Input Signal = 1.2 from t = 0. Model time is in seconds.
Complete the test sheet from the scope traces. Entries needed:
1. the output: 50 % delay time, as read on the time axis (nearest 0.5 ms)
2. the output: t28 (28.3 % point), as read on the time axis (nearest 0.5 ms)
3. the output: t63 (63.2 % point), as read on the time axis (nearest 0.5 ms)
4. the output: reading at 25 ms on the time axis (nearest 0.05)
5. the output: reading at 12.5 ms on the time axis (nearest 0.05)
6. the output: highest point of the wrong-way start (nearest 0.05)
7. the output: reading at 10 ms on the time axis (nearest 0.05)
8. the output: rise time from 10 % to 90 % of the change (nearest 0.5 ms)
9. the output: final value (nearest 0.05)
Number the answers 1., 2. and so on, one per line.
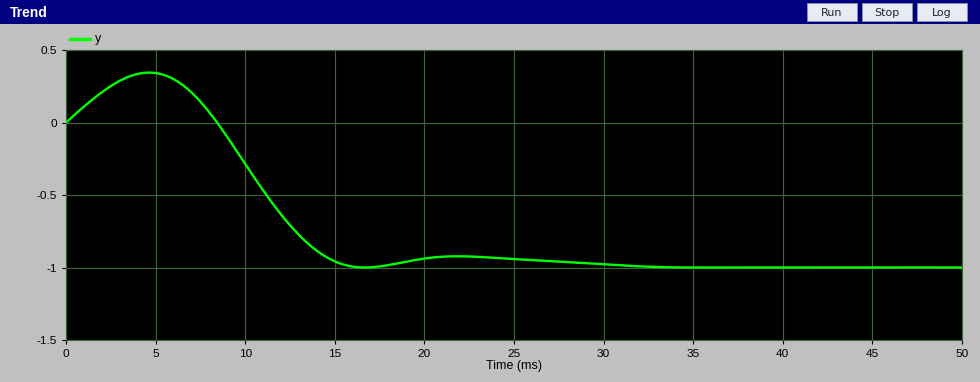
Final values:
1. 11.0 ms
2. 10.0 ms
3. 12.0 ms
4. -0.95
5. -0.70
6. 0.35
7. -0.30
8. 5.0 ms
9. -1.00
